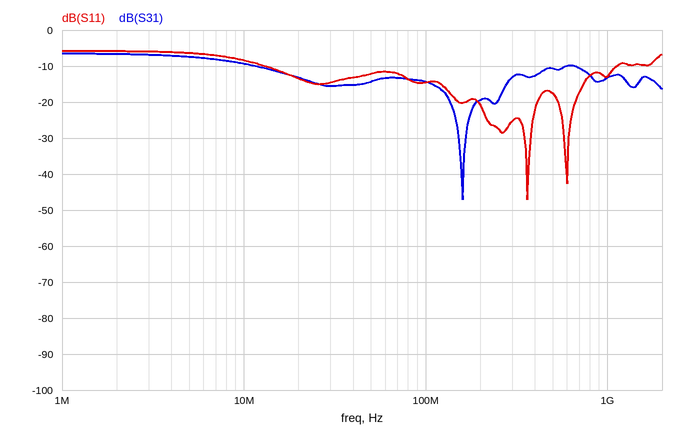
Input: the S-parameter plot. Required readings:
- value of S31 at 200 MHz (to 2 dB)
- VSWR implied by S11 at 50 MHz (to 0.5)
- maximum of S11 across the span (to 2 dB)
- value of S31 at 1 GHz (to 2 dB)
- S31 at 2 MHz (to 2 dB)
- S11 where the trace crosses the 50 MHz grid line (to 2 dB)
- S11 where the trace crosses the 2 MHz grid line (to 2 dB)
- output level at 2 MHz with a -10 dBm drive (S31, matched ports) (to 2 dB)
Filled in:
-20 dB
1.5
-6 dB
-14 dB
-6 dB
-12 dB
-6 dB
-16 dBm
